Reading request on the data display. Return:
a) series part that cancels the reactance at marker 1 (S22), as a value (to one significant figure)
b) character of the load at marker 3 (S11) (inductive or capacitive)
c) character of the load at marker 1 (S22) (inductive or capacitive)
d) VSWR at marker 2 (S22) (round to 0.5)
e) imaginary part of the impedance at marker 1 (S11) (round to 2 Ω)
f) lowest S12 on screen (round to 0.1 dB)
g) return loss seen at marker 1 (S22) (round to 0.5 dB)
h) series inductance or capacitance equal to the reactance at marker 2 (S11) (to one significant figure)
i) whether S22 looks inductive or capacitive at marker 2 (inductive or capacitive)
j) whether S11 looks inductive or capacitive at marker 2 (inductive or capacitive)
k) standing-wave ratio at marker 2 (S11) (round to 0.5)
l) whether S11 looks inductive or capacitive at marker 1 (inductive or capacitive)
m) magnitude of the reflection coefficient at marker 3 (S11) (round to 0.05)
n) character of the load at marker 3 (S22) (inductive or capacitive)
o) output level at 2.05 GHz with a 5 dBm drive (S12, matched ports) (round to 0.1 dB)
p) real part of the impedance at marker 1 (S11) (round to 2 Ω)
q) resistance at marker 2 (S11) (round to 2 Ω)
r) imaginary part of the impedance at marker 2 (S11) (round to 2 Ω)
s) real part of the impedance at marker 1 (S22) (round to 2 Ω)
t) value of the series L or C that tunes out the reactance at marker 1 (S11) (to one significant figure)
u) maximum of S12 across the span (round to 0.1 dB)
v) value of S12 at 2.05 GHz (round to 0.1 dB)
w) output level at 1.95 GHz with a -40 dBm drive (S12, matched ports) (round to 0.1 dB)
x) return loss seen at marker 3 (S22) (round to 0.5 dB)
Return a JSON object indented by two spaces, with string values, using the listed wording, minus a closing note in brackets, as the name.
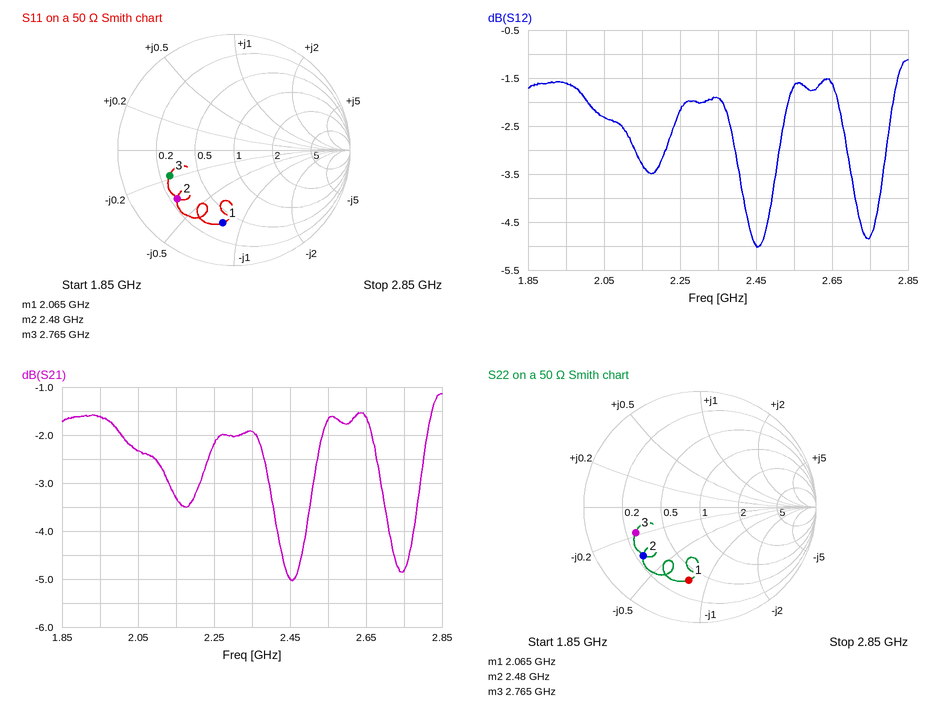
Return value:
{
  "series part that cancels the reactance at marker 1 (S22), as a value": "3 nH",
  "character of the load at marker 3 (S11)": "capacitive",
  "character of the load at marker 1 (S22)": "capacitive",
  "VSWR at marker 2 (S22)": "4.5",
  "imaginary part of the impedance at marker 1 (S11)": "-40 Ω",
  "lowest S12 on screen": "-5.0 dB",
  "return loss seen at marker 1 (S22)": "4.0 dB",
  "series inductance or capacitance equal to the reactance at marker 2 (S11)": "4 pF",
  "whether S22 looks inductive or capacitive at marker 2": "capacitive",
  "whether S11 looks inductive or capacitive at marker 2": "capacitive",
  "standing-wave ratio at marker 2 (S11)": "4.5",
  "whether S11 looks inductive or capacitive at marker 1": "capacitive",
  "magnitude of the reflection coefficient at marker 3 (S11)": "0.60",
  "character of the load at marker 3 (S22)": "capacitive",
  "output level at 2.05 GHz with a 5 dBm drive (S12, matched ports)": "2.7 dBm",
  "real part of the impedance at marker 1 (S11)": "18 Ω",
  "resistance at marker 2 (S11)": "12 Ω",
  "imaginary part of the impedance at marker 2 (S11)": "-18 Ω",
  "real part of the impedance at marker 1 (S22)": "18 Ω",
  "value of the series L or C that tunes out the reactance at marker 1 (S11)": "3 nH",
  "maximum of S12 across the span": "-1.1 dB",
  "value of S12 at 2.05 GHz": "-2.3 dB",
  "output level at 1.95 GHz with a -40 dBm drive (S12, matched ports)": "-41.6 dBm",
  "return loss seen at marker 3 (S22)": "4.5 dB"
}
